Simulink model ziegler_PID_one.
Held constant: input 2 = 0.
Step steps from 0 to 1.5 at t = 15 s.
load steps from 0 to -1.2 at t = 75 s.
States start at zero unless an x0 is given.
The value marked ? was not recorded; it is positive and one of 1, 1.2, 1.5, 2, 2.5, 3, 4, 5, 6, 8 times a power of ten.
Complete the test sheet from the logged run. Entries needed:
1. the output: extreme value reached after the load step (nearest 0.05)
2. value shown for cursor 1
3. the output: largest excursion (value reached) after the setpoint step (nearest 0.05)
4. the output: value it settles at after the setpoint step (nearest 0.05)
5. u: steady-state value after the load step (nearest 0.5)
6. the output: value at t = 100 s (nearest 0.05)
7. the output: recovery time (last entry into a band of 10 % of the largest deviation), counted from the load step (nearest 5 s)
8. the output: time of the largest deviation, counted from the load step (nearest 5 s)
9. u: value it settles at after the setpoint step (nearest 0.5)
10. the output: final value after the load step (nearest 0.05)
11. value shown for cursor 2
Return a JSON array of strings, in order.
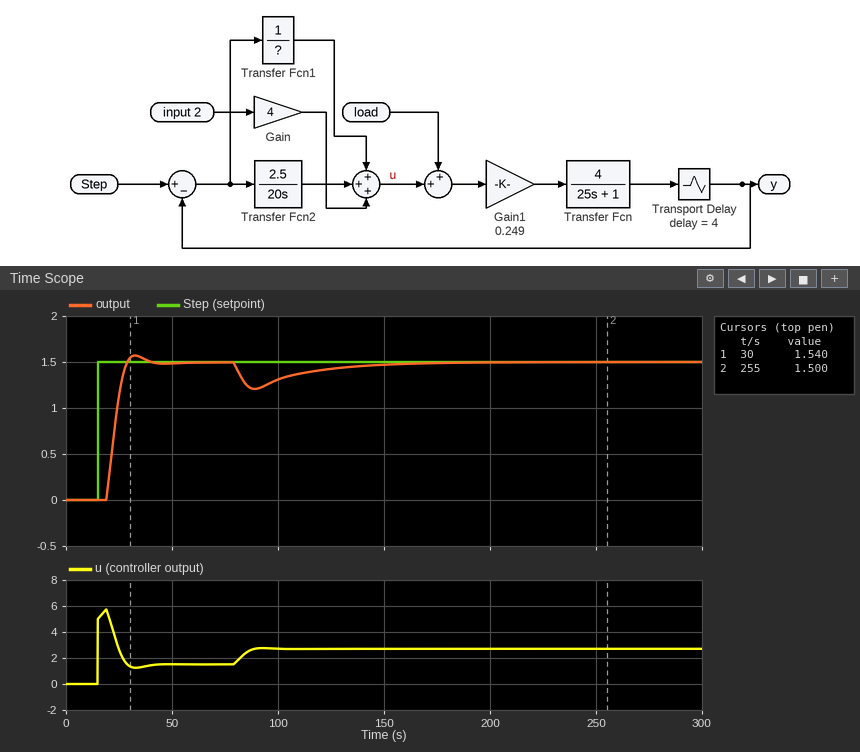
["1.20", "1.540", "1.55", "1.50", "2.5", "1.30", "75 s", "15 s", "1.5", "1.50", "1.500"]
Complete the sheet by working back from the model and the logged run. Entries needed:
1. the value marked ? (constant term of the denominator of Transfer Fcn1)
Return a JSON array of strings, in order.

["0.3"]
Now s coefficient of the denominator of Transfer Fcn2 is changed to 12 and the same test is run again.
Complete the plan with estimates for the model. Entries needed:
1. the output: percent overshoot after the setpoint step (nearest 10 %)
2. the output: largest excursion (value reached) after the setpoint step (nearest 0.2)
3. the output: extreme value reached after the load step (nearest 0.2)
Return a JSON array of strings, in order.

["20 %", "1.8", "1.2"]
